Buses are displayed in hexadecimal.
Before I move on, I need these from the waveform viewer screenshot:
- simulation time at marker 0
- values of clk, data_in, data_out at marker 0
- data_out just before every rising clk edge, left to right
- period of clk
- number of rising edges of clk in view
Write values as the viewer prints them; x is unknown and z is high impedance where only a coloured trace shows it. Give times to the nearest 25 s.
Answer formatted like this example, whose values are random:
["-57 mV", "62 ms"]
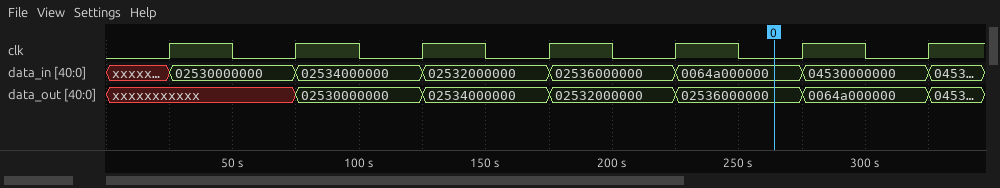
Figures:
["275 s", "clk=0, data_in=0064a000000, data_out=02536000000", "xxxxxxxxxxx, xxxxxxxxxxx, 02530000000, 02534000000, 02532000000, 02536000000, 0064a000000", "50 s", "7"]
